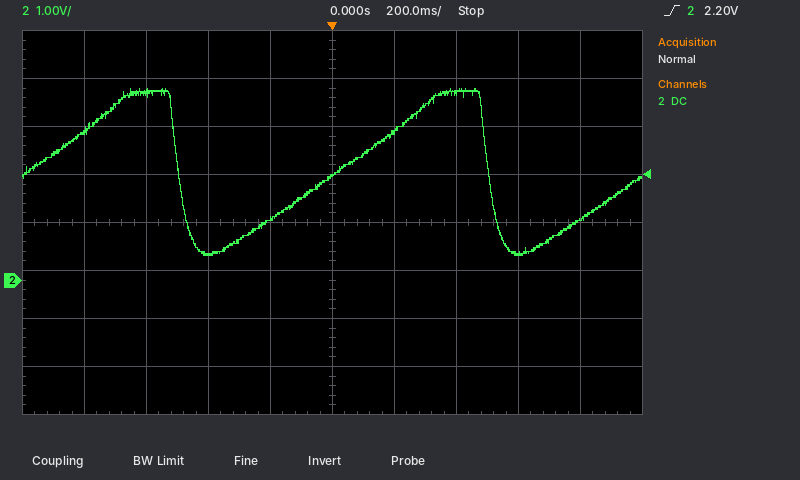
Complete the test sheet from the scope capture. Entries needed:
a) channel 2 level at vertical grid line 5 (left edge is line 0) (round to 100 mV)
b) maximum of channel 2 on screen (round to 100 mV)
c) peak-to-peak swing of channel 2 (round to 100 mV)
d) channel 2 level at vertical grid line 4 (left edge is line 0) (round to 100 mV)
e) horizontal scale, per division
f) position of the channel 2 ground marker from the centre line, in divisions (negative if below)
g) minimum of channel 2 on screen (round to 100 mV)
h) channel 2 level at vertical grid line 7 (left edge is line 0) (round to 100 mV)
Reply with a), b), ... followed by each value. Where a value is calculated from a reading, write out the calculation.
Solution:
a) 2.2 V
b) 4.0 V
c) 4.0 V − (500 mV) = 3.5 V
d) 1.3 V
e) 200 ms
f) -1.2 div
g) 500 mV
h) 3.9 V
